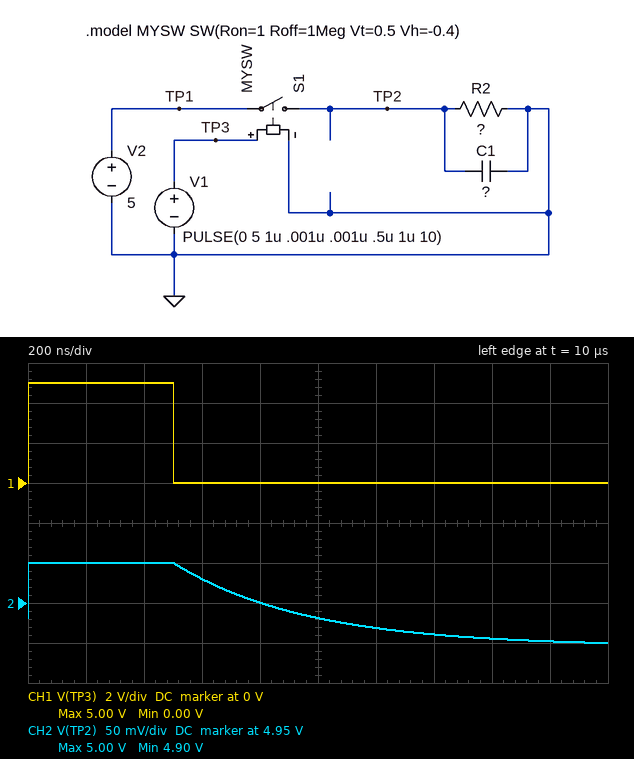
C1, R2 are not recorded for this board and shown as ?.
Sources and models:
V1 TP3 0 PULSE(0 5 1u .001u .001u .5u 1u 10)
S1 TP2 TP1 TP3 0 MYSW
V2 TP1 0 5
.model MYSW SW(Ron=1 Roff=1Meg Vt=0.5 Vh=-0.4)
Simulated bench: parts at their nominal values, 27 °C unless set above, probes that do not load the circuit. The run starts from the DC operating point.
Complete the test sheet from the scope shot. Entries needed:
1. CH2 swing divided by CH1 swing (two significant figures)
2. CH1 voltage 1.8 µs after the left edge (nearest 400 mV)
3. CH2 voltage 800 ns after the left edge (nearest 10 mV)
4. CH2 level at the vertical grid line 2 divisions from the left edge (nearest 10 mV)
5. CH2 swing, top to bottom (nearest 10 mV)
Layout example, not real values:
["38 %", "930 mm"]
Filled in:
["0.020", "0 V", "4.95 V", "5.00 V", "100 mV"]
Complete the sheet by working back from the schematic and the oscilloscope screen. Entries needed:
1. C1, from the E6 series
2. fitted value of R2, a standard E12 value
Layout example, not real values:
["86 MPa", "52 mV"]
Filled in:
["470 fF", "47 MΩ"]
